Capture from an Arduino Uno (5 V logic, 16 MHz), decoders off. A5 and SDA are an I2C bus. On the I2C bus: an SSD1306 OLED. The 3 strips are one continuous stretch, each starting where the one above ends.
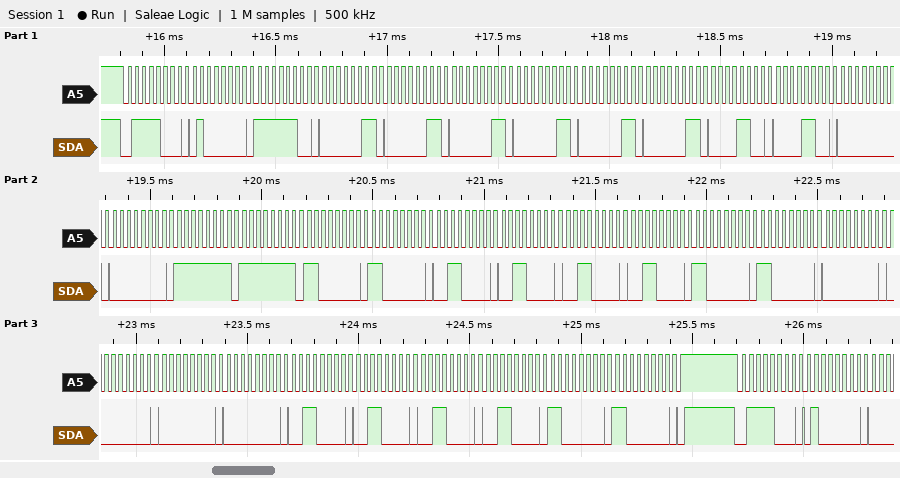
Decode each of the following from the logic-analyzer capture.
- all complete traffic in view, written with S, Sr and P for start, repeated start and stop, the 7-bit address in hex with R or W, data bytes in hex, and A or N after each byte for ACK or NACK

S 3CW A 40 A FC A 03 A 03 A 03 A 03 A 03 A 03 A 0C A 0C A 00 A 00 A FF A FF A C0 A C0 A 30 A 30 A 30 A 30 A C0 A C0 A 00 A 00 A 00 A 00 A 30 A 30 A 30 A 30 A C0 A C0 A P S 3CW A 40 A
